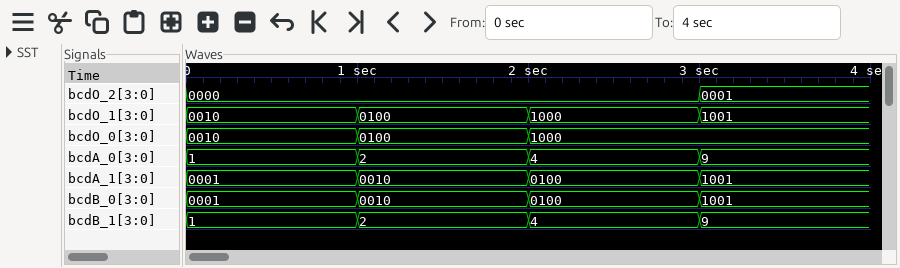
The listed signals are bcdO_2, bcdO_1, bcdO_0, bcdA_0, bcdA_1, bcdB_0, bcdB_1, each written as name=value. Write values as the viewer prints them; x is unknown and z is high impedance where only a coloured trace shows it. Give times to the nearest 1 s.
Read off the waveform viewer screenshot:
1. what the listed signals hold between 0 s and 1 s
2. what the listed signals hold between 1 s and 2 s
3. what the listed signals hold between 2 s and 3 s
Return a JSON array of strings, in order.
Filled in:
["bcdO_2=0000, bcdO_1=0010, bcdO_0=0010, bcdA_0=1, bcdA_1=0001, bcdB_0=0001, bcdB_1=1", "bcdO_2=0000, bcdO_1=0100, bcdO_0=0100, bcdA_0=2, bcdA_1=0010, bcdB_0=0010, bcdB_1=2", "bcdO_2=0000, bcdO_1=1000, bcdO_0=1000, bcdA_0=4, bcdA_1=0100, bcdB_0=0100, bcdB_1=4"]
